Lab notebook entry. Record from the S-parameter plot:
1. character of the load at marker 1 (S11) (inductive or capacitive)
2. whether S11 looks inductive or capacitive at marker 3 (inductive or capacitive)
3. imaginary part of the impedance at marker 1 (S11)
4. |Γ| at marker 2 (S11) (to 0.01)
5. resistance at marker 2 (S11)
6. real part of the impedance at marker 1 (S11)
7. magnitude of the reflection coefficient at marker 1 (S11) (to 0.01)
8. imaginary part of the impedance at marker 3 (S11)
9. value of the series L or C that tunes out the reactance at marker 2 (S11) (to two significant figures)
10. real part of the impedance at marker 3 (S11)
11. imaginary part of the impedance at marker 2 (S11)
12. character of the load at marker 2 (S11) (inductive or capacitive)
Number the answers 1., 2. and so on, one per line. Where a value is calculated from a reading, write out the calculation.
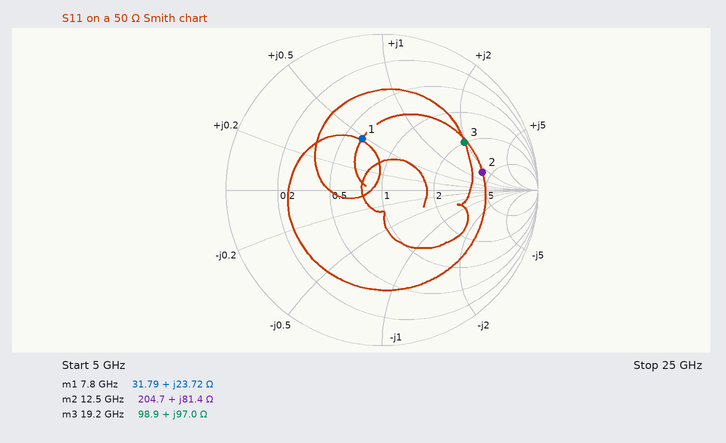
1. inductive
2. inductive
3. +23.72 Ω
4. 0.65
5. 204.7 Ω
6. 31.79 Ω
7. 0.35
8. +97.0 Ω
9. C = 1/(2π × 12.5 GHz × 81.4 Ω) ≈ 156 fF, so 160 fF to two significant figures
10. 98.9 Ω
11. +81.4 Ω
12. inductive
